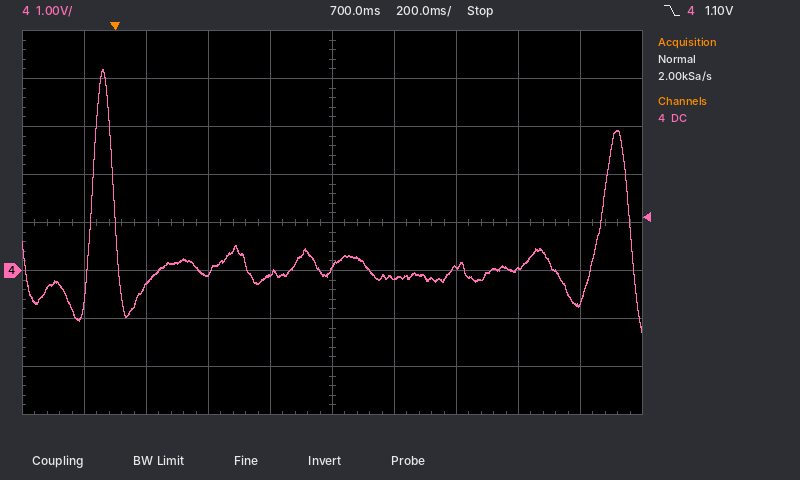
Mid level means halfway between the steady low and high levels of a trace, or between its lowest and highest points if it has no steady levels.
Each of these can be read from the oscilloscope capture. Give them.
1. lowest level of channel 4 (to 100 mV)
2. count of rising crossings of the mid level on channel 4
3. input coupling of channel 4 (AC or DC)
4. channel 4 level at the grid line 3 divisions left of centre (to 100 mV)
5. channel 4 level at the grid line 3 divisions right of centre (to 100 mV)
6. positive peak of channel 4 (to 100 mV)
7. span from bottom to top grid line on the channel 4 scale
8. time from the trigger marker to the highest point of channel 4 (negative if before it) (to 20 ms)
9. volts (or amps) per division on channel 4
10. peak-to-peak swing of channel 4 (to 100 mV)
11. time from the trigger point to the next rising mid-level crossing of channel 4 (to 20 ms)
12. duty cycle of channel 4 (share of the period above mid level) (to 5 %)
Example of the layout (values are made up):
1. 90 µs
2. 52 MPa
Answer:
1. -1.3 V
2. 2
3. DC
4. -300 mV
5. 0.0 V
6. 4.2 V
7. 8 V
8. -40 ms
9. 1 V
10. 5.5 V
11. 1.58 s
12. 5 %
